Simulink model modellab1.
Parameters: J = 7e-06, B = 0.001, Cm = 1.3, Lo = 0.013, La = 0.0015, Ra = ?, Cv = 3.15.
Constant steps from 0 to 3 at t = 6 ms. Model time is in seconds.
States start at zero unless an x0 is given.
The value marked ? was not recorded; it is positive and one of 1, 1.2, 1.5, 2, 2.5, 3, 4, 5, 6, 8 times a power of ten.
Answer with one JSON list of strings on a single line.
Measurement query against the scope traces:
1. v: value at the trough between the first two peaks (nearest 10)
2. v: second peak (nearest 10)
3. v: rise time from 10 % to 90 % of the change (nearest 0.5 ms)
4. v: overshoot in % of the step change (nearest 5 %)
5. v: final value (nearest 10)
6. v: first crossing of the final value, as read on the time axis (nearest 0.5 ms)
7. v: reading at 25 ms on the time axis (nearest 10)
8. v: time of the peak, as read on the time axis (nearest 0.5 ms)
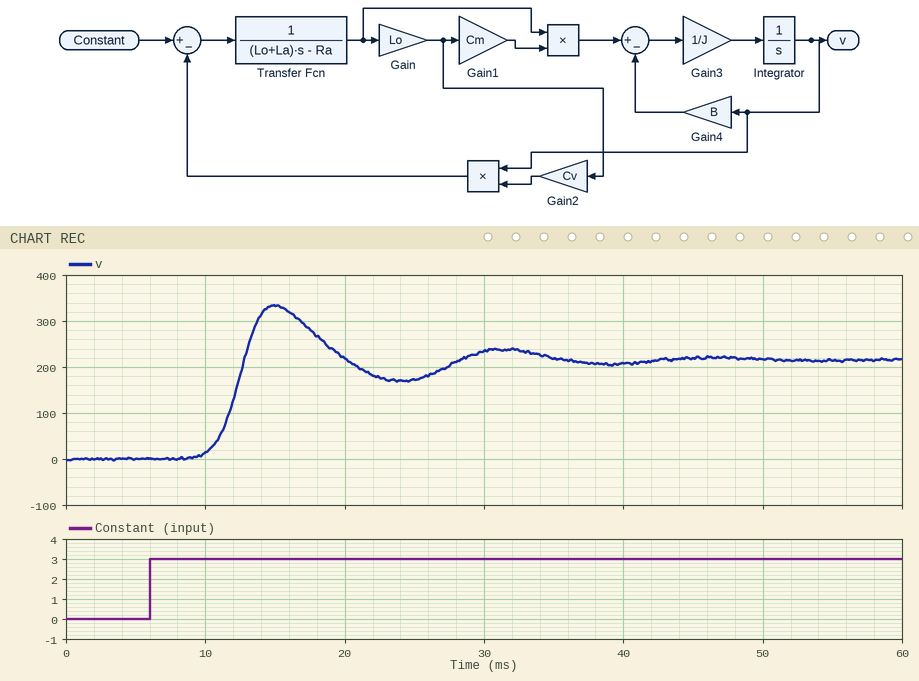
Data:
["170", "240", "2.5 ms", "55 %", "220", "13.0 ms", "170", "15.0 ms"]
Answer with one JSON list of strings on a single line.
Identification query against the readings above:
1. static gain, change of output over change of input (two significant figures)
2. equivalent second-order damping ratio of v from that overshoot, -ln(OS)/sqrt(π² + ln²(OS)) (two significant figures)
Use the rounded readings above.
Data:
["73", "0.19"]
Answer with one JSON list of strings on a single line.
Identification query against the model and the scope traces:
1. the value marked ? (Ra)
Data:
["8"]
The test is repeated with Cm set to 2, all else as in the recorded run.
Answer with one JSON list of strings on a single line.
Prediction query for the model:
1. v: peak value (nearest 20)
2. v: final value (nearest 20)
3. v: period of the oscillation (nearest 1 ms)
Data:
["340", "220", "16 ms"]
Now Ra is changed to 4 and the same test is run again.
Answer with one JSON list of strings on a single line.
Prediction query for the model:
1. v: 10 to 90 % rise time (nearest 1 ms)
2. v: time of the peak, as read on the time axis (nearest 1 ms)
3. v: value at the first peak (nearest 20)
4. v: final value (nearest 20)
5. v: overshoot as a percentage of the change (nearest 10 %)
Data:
["4 ms", "18 ms", "180", "120", "40 %"]
